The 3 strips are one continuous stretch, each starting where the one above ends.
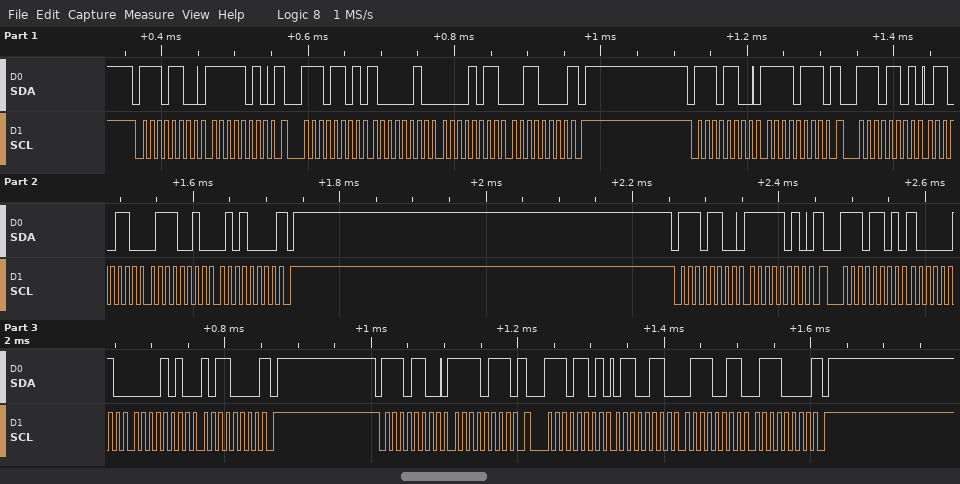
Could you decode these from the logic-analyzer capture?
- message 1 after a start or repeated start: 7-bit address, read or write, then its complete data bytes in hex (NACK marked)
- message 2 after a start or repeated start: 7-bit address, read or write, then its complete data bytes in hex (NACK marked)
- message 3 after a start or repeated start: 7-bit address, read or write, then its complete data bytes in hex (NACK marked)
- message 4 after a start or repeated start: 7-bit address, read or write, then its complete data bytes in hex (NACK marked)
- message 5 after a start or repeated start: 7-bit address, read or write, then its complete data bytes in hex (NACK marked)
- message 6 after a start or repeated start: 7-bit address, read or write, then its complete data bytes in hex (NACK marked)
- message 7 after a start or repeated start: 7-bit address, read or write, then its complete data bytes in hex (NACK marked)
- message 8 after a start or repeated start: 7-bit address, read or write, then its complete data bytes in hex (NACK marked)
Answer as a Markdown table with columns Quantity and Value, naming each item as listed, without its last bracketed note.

| Quantity | Value |
|---|---|
| message 1 after a start or repeated start: 7-bit address, read or write, then its complete data bytes in hex | 0x76 write: FA |
| message 2 after a start or repeated start: 7-bit address, read or write, then its complete data bytes in hex | 0x76 read: 82 0B 30 NACK |
| message 3 after a start or repeated start: 7-bit address, read or write, then its complete data bytes in hex | 0x76 write: F7 |
| message 4 after a start or repeated start: 7-bit address, read or write, then its complete data bytes in hex | 0x76 read: 66 72 50 NACK |
| message 5 after a start or repeated start: 7-bit address, read or write, then its complete data bytes in hex | 0x76 write: FA |
| message 6 after a start or repeated start: 7-bit address, read or write, then its complete data bytes in hex | 0x76 read: 82 0A B0 NACK |
| message 7 after a start or repeated start: 7-bit address, read or write, then its complete data bytes in hex | 0x76 write: F7 |
| message 8 after a start or repeated start: 7-bit address, read or write, then its complete data bytes in hex | 0x76 read: 66 73 70 NACK |
